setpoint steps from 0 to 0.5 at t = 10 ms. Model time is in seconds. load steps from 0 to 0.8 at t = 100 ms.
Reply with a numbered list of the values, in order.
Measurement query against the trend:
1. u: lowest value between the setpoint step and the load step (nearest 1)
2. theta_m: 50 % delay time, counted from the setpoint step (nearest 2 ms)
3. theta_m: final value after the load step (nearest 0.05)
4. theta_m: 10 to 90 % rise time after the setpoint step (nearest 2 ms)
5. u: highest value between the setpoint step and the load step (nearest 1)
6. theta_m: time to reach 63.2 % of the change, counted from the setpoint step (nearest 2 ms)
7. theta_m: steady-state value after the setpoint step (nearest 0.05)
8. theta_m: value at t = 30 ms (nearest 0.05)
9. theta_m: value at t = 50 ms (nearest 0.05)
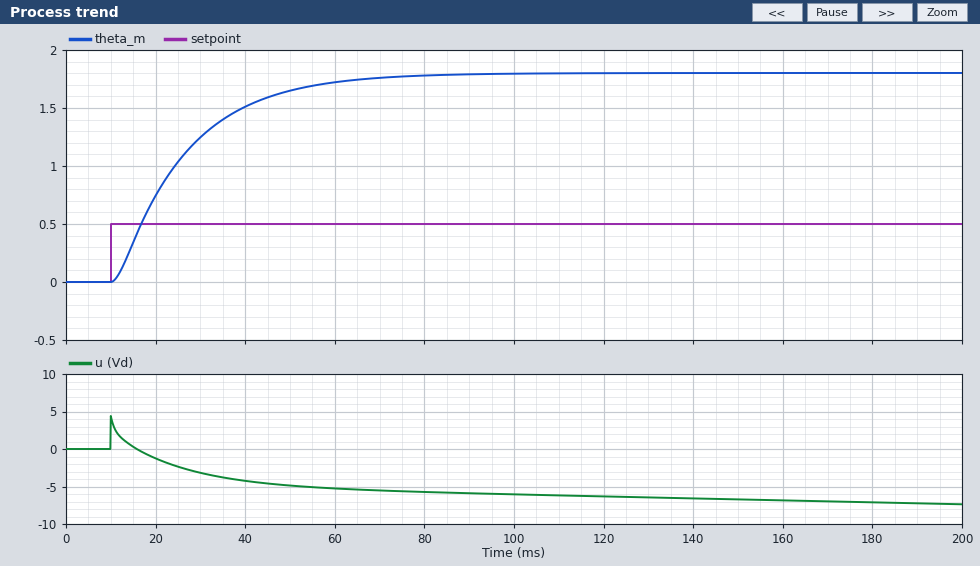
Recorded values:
1. -6
2. 12 ms
3. 1.80
4. 34 ms
5. 4
6. 18 ms
7. 1.80
8. 1.25
9. 1.65
